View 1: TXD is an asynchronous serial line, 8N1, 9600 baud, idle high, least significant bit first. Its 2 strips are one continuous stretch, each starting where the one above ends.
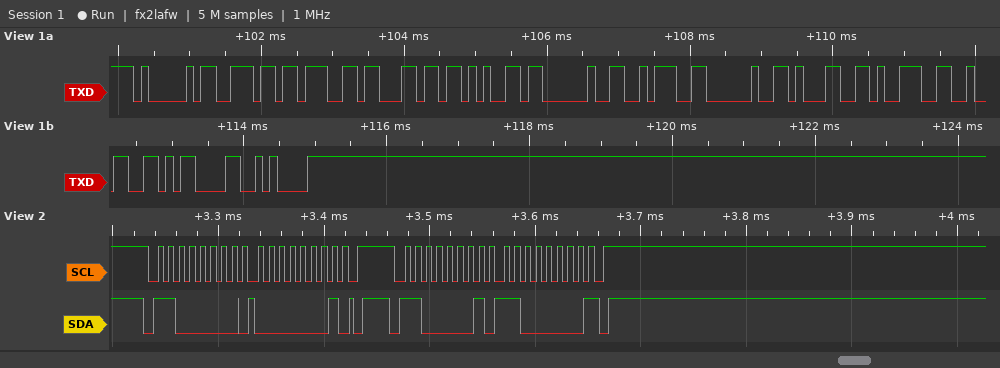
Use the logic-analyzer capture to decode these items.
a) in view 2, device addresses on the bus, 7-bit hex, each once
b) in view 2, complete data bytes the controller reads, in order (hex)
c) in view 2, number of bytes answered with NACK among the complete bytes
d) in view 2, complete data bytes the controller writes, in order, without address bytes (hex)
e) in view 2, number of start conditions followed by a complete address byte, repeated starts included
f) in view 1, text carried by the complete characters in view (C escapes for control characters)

0x60
C0
1
01
2
"Angle : 192\r\n"
